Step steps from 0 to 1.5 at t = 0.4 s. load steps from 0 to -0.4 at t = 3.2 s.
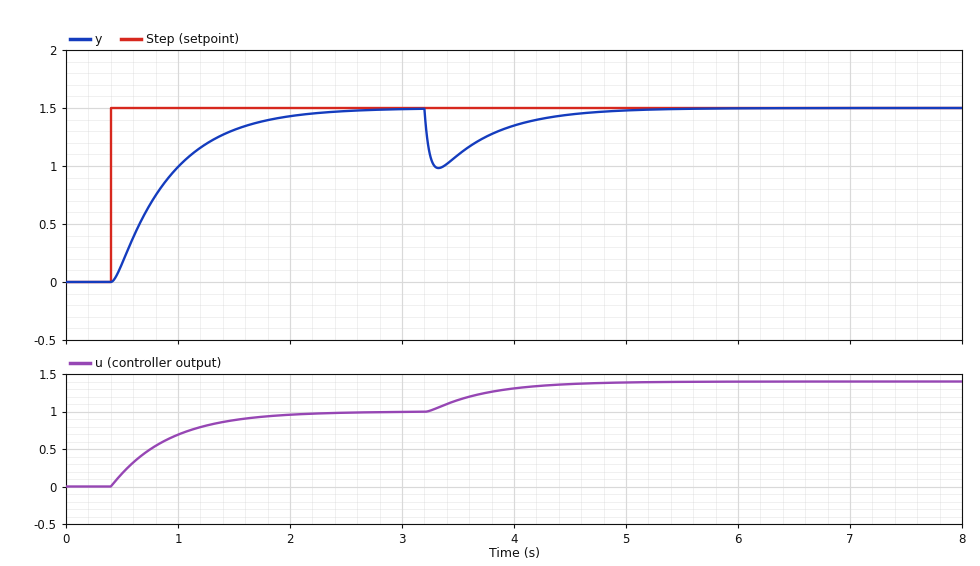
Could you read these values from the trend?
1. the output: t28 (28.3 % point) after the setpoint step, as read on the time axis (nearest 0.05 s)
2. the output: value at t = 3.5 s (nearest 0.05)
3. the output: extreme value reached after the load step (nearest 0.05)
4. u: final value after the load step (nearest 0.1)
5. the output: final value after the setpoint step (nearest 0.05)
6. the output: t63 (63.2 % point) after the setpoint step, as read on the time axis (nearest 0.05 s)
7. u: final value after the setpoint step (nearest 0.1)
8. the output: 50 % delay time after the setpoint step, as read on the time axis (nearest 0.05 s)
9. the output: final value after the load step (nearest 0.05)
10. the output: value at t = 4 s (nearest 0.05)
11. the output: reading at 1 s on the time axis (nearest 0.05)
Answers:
0.60 s
1.10
1.00
1.4
1.50
0.95 s
1.0
0.80 s
1.50
1.35
1.00
